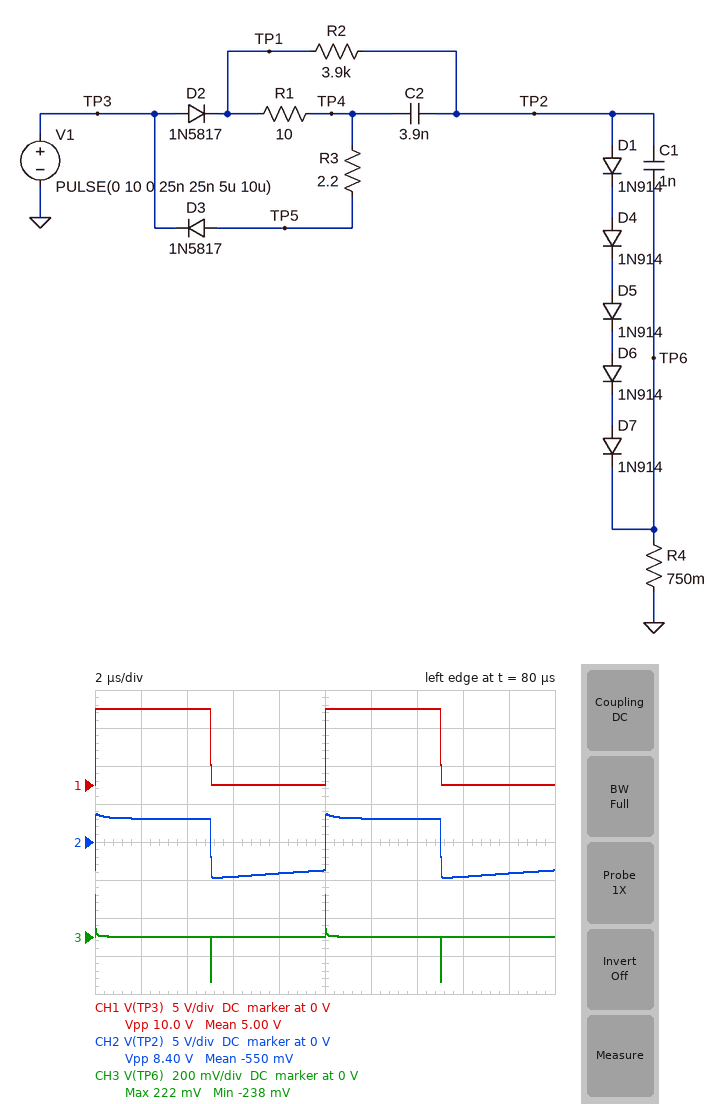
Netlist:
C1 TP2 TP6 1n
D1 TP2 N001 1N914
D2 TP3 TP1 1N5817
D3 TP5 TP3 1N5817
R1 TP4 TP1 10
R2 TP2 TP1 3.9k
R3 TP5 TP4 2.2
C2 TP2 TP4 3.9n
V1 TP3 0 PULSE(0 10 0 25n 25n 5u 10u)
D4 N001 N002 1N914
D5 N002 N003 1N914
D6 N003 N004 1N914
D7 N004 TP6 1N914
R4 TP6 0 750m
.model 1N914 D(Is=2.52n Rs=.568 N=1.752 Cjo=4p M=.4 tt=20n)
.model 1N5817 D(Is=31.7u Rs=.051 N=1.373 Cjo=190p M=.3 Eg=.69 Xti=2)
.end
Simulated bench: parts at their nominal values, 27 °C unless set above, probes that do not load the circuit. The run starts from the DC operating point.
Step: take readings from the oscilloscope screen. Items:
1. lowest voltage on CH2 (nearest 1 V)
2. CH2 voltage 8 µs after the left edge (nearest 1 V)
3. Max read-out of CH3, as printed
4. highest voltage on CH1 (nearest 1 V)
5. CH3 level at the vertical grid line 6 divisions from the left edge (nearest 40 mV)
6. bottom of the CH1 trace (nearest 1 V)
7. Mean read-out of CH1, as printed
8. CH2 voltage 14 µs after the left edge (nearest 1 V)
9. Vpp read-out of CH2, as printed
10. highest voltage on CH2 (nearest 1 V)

-5 V
-4 V
222 mV
10 V
0 V
0 V
5.00 V
3 V
8.40 V
4 V
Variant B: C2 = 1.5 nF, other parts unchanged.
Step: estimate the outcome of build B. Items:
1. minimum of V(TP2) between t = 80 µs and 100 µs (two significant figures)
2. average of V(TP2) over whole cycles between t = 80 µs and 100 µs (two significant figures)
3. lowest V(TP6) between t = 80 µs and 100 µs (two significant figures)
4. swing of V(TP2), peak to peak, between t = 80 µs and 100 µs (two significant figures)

-2.8 V
430 mV
-180 mV
6.5 V
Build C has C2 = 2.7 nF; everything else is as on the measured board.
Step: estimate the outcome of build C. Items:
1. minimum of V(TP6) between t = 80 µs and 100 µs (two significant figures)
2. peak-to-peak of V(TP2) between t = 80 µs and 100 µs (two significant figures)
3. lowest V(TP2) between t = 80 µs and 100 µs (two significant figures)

-220 mV
7.8 V
-4.0 V
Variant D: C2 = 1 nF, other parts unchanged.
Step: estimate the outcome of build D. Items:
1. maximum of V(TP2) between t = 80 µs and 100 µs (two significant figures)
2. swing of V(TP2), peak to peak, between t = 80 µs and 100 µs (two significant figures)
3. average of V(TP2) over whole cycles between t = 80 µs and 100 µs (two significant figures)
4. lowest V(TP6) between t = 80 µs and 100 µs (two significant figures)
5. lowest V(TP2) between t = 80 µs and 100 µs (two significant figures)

3.6 V
5.4 V
850 mV
-150 mV
-1.8 V
